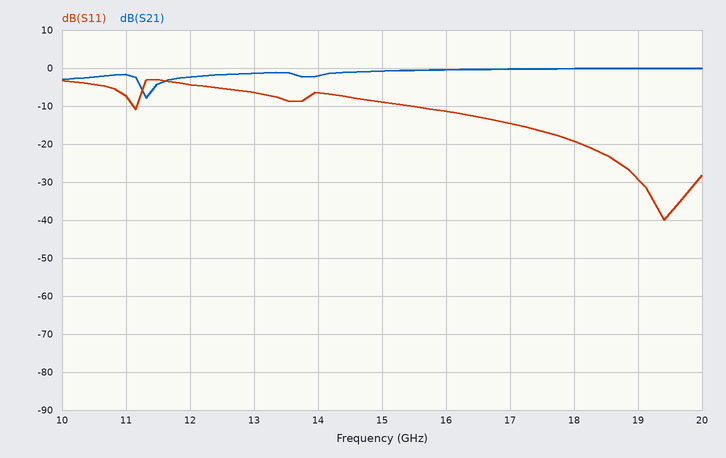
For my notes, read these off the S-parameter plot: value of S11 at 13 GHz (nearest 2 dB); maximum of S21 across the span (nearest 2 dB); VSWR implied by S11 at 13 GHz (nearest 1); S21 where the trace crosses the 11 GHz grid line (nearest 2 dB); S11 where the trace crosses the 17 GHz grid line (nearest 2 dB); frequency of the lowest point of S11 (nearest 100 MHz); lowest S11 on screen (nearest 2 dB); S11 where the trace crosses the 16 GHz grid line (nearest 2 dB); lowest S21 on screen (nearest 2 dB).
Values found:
-6 dB
0 dB
3
-2 dB
-14 dB
19.4 GHz
-40 dB
-12 dB
-8 dB
